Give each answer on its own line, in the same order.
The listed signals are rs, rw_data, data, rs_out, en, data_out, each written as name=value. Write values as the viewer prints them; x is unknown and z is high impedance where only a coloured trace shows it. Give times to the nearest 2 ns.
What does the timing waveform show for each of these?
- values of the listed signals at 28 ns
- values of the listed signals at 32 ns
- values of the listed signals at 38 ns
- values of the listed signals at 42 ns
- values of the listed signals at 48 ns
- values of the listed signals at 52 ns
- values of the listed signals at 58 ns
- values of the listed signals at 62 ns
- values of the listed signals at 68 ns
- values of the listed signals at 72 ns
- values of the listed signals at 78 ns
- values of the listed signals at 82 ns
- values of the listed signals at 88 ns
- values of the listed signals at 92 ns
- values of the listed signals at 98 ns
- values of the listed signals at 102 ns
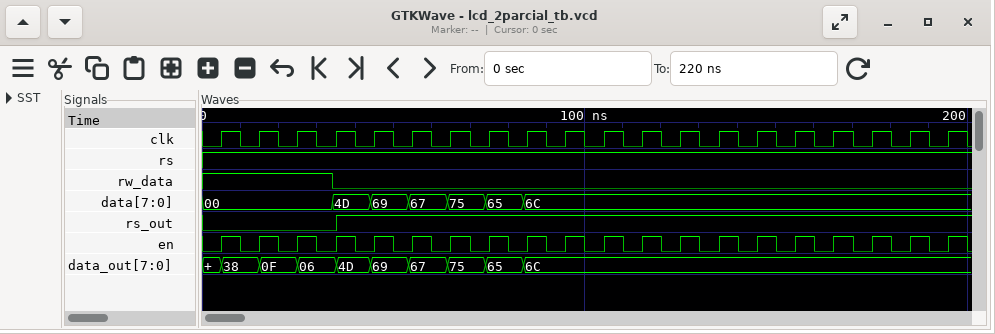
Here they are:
rs=1, rw_data=1, data=00, rs_out=0, en=1, data_out=06
rs=1, rw_data=1, data=00, rs_out=0, en=0, data_out=06
rs=1, rw_data=0, data=4D, rs_out=1, en=1, data_out=4D
rs=1, rw_data=0, data=4D, rs_out=1, en=0, data_out=4D
rs=1, rw_data=0, data=69, rs_out=1, en=1, data_out=69
rs=1, rw_data=0, data=69, rs_out=1, en=0, data_out=69
rs=1, rw_data=0, data=67, rs_out=1, en=1, data_out=67
rs=1, rw_data=0, data=67, rs_out=1, en=0, data_out=67
rs=1, rw_data=0, data=75, rs_out=1, en=1, data_out=75
rs=1, rw_data=0, data=75, rs_out=1, en=0, data_out=75
rs=1, rw_data=0, data=65, rs_out=1, en=1, data_out=65
rs=1, rw_data=0, data=65, rs_out=1, en=0, data_out=65
rs=1, rw_data=0, data=6C, rs_out=1, en=1, data_out=6C
rs=1, rw_data=0, data=6C, rs_out=1, en=0, data_out=6C
rs=1, rw_data=0, data=6C, rs_out=1, en=1, data_out=6C
rs=1, rw_data=0, data=6C, rs_out=1, en=0, data_out=6C
